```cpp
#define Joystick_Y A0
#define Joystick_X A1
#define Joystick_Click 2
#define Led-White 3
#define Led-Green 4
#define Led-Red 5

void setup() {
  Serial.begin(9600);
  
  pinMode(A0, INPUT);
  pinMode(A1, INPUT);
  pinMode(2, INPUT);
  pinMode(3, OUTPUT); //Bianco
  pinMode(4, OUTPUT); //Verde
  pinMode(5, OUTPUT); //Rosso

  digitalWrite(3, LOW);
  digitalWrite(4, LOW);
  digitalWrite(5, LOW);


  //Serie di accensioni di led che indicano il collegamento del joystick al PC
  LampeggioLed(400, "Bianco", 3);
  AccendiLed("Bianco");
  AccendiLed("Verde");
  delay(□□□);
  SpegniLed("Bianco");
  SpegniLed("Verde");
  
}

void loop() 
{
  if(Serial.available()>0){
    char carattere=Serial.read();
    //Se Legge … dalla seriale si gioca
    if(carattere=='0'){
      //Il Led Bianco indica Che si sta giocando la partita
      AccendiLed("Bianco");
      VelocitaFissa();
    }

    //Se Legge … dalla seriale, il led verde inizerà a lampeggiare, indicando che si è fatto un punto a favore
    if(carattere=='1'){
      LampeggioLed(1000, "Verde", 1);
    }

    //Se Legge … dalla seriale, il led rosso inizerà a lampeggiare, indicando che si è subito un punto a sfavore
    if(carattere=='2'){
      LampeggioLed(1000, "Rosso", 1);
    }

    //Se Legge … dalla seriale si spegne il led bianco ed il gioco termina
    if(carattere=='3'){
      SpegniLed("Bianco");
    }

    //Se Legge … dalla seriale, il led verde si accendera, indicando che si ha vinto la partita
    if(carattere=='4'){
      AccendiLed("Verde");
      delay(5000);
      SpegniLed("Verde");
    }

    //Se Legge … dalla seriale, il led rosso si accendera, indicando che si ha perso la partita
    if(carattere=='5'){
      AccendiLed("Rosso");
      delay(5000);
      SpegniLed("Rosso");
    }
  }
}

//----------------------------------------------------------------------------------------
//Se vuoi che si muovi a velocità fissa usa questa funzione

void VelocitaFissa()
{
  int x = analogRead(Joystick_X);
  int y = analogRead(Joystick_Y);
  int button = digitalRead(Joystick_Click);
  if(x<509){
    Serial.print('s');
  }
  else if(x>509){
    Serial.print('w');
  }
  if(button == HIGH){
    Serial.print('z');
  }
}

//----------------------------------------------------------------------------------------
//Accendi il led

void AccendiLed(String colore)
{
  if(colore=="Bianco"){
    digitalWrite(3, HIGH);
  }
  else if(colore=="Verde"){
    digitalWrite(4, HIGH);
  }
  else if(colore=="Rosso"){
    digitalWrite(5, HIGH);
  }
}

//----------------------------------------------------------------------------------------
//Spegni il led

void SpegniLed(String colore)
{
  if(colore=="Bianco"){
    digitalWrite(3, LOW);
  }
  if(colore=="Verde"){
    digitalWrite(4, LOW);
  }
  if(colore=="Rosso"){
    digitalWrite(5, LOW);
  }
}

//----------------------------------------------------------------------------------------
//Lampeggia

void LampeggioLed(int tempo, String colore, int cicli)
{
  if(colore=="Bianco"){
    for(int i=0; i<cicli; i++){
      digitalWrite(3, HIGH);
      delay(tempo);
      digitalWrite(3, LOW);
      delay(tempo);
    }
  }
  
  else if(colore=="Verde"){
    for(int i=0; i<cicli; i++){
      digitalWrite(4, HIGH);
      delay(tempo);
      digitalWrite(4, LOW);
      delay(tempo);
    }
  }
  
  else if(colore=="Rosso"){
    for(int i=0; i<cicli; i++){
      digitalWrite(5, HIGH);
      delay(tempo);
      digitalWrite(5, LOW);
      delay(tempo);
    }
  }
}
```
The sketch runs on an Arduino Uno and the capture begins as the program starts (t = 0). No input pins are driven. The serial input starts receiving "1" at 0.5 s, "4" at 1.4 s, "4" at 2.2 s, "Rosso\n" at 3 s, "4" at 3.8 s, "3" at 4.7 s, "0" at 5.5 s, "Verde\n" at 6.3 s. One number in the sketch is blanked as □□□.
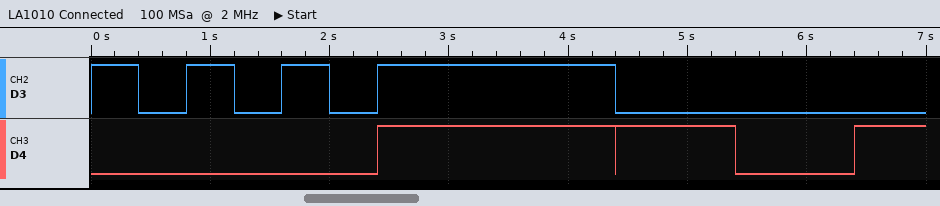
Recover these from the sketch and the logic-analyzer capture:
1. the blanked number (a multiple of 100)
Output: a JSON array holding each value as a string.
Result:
["2000"]
